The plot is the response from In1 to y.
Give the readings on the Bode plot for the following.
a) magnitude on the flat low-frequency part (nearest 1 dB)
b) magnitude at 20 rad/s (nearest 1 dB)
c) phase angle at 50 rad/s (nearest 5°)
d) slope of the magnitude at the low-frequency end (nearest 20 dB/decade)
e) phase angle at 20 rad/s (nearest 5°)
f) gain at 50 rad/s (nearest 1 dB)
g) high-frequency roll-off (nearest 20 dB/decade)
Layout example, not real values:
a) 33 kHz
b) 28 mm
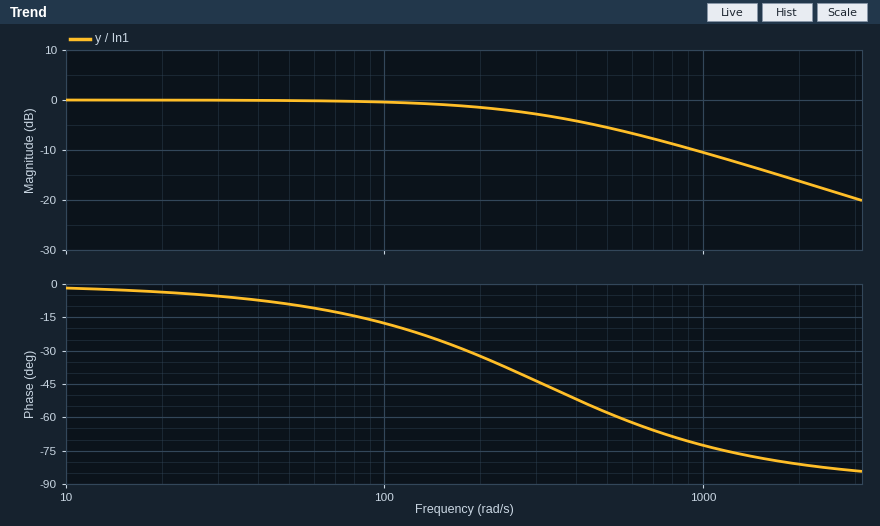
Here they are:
a) 0 dB
b) 0 dB
c) -10°
d) 0 dB/decade
e) -5°
f) 0 dB
g) -20 dB/decade
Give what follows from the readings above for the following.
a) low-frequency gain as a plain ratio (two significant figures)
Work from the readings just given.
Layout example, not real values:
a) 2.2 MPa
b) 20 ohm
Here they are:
a) 1.0
